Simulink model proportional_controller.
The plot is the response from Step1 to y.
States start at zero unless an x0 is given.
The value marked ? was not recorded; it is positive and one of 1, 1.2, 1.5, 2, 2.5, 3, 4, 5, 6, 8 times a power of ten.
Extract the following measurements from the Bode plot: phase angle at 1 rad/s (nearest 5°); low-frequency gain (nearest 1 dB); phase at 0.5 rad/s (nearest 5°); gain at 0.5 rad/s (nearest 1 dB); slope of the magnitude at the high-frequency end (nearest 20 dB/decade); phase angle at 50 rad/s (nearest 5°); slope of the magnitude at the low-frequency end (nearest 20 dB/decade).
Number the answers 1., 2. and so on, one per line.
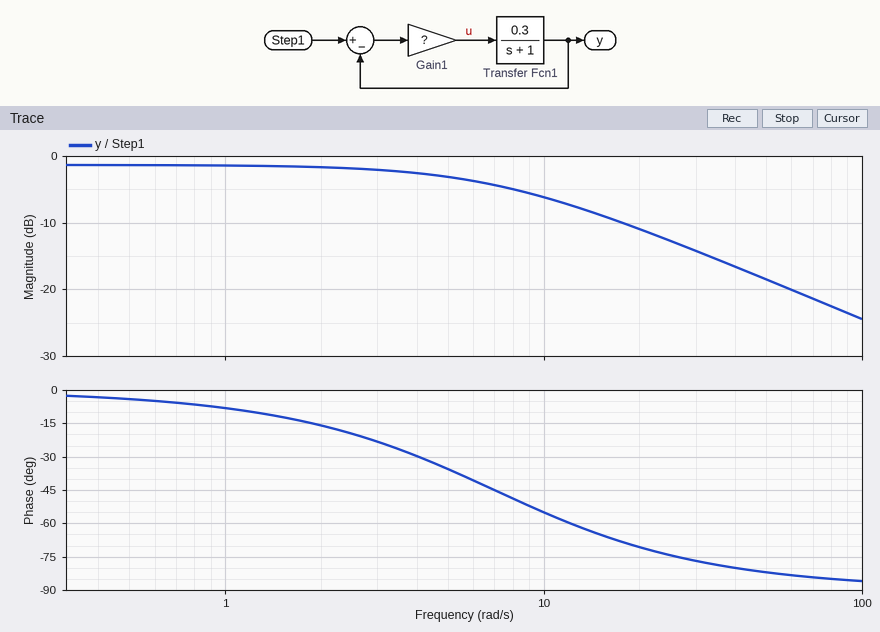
1. -10°
2. -1 dB
3. -5°
4. -1 dB
5. -20 dB/decade
6. -80°
7. 0 dB/decade
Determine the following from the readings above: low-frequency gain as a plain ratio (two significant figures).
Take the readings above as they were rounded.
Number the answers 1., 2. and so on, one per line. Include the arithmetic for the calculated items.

1. 10^(-1 / 20) = 0.89
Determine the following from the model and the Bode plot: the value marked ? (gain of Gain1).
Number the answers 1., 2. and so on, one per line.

1. 20
